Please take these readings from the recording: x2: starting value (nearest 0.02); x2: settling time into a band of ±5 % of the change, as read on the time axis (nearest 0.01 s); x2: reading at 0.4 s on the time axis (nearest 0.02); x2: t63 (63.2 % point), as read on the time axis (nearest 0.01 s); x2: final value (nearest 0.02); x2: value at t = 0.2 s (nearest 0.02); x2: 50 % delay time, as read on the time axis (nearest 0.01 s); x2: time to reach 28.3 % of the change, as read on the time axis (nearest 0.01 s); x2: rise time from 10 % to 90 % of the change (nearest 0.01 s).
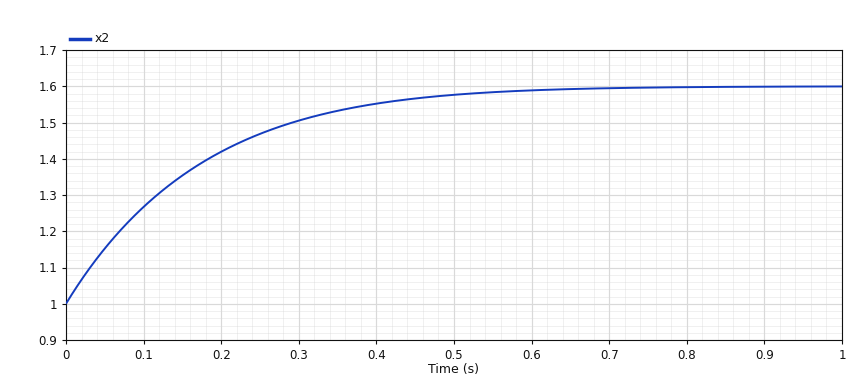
1.00
0.47 s
1.56
0.17 s
1.60
1.42
0.12 s
0.06 s
0.35 s
